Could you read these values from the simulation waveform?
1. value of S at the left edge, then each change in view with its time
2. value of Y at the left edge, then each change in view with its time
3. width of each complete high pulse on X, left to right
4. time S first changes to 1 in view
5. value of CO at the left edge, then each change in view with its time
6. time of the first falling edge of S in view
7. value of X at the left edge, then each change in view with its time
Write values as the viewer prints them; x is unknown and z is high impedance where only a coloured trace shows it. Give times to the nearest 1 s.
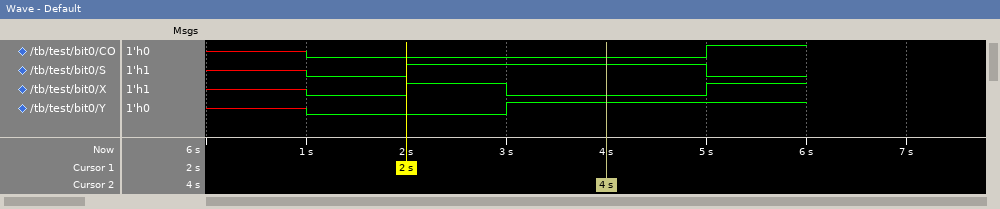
x, 0 at 1 s, 1 at 2 s, 0 at 5 s
x, 0 at 1 s, 1 at 3 s
1 s
2 s
x, 0 at 1 s, 1 at 5 s
5 s
x, 0 at 1 s, 1 at 2 s, 0 at 3 s, 1 at 5 s
